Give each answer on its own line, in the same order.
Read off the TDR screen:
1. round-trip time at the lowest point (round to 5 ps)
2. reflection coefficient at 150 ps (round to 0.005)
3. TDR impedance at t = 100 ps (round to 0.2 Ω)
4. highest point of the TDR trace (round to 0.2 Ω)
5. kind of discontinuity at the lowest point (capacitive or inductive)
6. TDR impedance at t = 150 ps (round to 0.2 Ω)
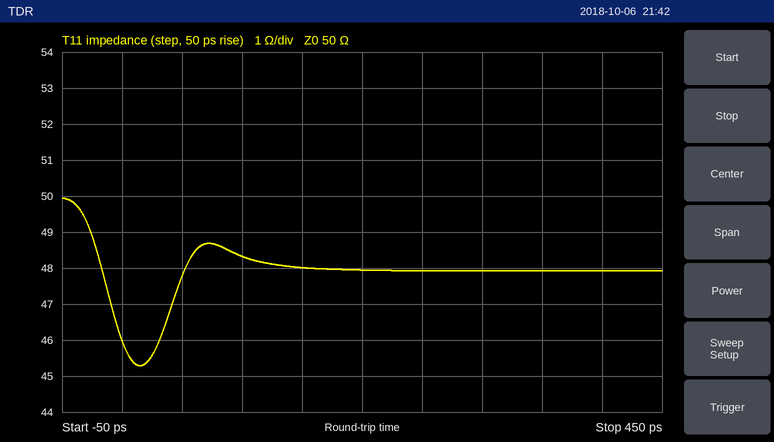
15 ps
-0.020
48.4 Ω
50.0 Ω
capacitive
48.0 Ω
